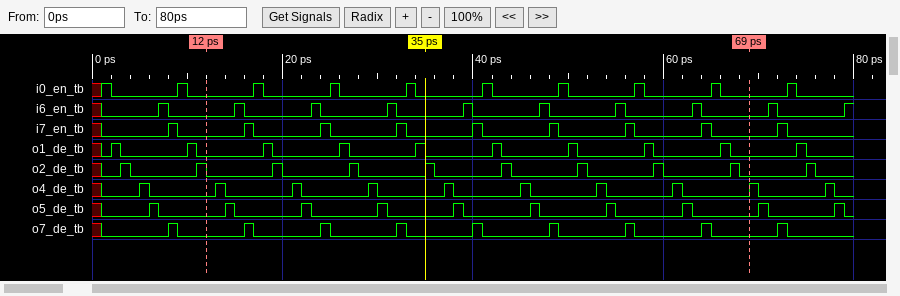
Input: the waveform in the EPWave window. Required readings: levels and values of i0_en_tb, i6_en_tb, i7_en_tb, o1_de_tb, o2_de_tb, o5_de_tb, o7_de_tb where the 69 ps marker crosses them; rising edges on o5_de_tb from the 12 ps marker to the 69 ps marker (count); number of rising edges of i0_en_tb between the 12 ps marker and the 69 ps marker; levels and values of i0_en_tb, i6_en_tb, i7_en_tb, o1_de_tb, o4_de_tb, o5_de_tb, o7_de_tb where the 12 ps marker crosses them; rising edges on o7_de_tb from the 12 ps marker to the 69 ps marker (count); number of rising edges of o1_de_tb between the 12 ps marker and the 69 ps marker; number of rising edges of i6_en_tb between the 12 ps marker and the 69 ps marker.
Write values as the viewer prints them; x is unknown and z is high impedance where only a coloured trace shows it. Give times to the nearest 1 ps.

i0_en_tb=0, i6_en_tb=0, i7_en_tb=0, o1_de_tb=0, o2_de_tb=0, o5_de_tb=0, o7_de_tb=0
7
7
i0_en_tb=0, i6_en_tb=0, i7_en_tb=0, o1_de_tb=0, o4_de_tb=0, o5_de_tb=0, o7_de_tb=0
7
7
7
